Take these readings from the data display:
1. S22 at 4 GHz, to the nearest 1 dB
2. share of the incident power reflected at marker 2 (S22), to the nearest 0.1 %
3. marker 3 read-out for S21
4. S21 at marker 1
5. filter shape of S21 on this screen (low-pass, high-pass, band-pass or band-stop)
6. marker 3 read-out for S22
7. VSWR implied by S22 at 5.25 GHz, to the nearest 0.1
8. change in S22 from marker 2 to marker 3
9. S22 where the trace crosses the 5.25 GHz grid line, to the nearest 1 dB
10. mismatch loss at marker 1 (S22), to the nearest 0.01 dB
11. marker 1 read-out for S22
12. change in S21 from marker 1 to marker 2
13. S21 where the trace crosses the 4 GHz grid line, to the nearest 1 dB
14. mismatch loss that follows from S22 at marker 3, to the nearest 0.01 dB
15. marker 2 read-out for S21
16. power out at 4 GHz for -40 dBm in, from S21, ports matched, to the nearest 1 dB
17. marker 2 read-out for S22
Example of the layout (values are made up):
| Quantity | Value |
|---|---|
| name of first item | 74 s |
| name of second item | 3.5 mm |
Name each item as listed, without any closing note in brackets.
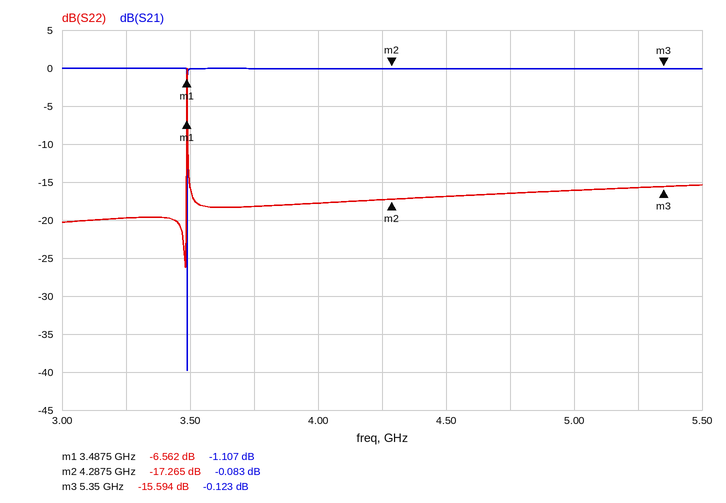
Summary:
| Quantity | Value |
|---|---|
| S22 at 4 GHz, to the nearest 1 dB | -18 dB |
| share of the incident power reflected at marker 2 (S22), to the nearest 0.1 % | 1.9 % |
| marker 3 read-out for S21 | -0.123 dB |
| S21 at marker 1 | -1.107 dB |
| filter shape of S21 on this screen | band-stop |
| marker 3 read-out for S22 | -15.594 dB |
| VSWR implied by S22 at 5.25 GHz, to the nearest 0.1 | 1.4 |
| change in S22 from marker 2 to marker 3 | 1.671 dB |
| S22 where the trace crosses the 5.25 GHz grid line, to the nearest 1 dB | -16 dB |
| mismatch loss at marker 1 (S22), to the nearest 0.01 dB | 1.08 dB |
| marker 1 read-out for S22 | -6.562 dB |
| change in S21 from marker 1 to marker 2 | 1.024 dB |
| S21 where the trace crosses the 4 GHz grid line, to the nearest 1 dB | 0 dB |
| mismatch loss that follows from S22 at marker 3, to the nearest 0.01 dB | 0.12 dB |
| marker 2 read-out for S21 | -0.083 dB |
| power out at 4 GHz for -40 dBm in, from S21, ports matched, to the nearest 1 dB | -40 dBm |
| marker 2 read-out for S22 | -17.265 dB |
